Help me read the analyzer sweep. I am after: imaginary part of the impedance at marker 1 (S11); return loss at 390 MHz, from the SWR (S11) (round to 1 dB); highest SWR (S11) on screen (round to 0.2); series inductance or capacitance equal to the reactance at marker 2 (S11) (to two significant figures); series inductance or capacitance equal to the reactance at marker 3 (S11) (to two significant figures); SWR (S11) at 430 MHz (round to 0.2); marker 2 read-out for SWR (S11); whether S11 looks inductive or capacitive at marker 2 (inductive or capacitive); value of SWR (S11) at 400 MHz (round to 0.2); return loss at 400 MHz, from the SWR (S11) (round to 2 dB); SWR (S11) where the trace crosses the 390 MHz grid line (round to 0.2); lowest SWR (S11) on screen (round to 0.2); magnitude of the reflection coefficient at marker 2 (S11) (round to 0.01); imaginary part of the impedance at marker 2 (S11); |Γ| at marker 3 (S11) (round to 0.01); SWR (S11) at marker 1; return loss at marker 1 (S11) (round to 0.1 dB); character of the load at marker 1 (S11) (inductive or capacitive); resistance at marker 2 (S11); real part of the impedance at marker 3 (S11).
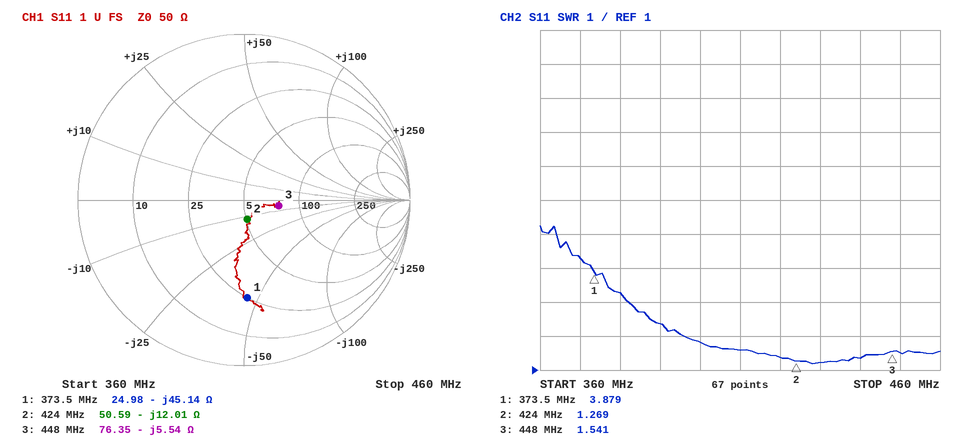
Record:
-45.14 Ω
8 dB
5.2
31 pF
64 pF
1.2
1.269
capacitive
1.8
10 dB
2.4
1.2
0.12
-12.01 Ω
0.21
3.879
4.6 dB
capacitive
50.59 Ω
76.35 Ω
